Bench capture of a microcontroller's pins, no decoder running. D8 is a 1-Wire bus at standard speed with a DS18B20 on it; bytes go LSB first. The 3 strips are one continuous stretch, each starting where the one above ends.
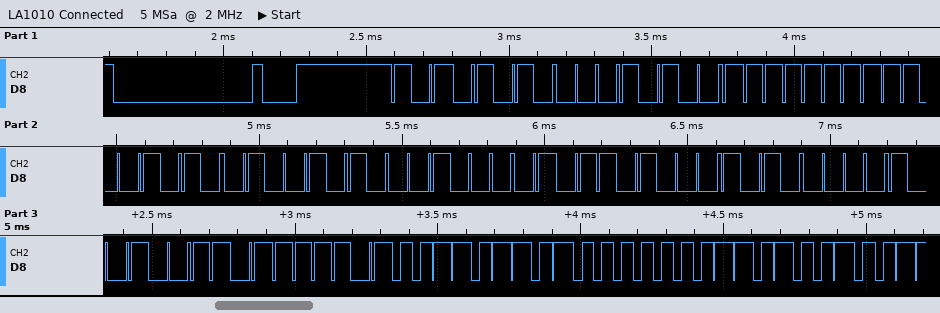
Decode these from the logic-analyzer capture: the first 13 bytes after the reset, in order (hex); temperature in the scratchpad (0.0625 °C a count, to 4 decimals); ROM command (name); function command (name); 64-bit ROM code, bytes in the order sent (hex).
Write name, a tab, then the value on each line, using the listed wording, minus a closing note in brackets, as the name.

the first 13 bytes after the reset, in order	55 28 FF 53 52 84 16 05 C9 BE 6C 01 4B
temperature in the scratchpad	22.7500 °C
ROM command	Match ROM
function command	Read Scratchpad
64-bit ROM code, bytes in the order sent	28 FF 53 52 84 16 05 C9
